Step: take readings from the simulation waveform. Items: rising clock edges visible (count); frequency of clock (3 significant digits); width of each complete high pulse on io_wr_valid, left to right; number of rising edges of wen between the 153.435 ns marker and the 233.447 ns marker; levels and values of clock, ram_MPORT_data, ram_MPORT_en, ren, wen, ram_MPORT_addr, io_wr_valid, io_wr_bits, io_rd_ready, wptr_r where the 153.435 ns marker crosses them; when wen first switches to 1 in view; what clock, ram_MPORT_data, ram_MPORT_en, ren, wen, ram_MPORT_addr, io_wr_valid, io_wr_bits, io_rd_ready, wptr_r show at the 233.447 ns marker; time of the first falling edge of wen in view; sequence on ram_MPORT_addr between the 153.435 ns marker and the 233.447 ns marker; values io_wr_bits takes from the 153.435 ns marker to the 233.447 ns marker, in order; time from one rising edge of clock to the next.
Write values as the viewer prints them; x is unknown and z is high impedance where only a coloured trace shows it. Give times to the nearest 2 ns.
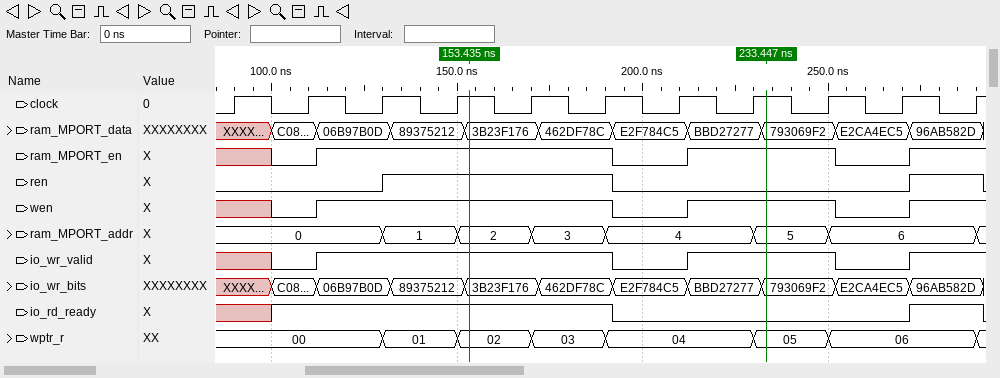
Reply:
11
50.0 MHz
80 ns, 40 ns
1
clock=1, ram_MPORT_data=3B23F176, ram_MPORT_en=1, ren=1, wen=1, ram_MPORT_addr=2, io_wr_valid=1, io_wr_bits=3B23F176, io_rd_ready=1, wptr_r=02
112 ns
clock=1, ram_MPORT_data=793069F2, ram_MPORT_en=1, ren=0, wen=1, ram_MPORT_addr=5, io_wr_valid=1, io_wr_bits=793069F2, io_rd_ready=0, wptr_r=05
192 ns
2, 3, 4, 5
3B23F176, 462DF78C, E2F784C5, BBD27277, 793069F2
20 ns
